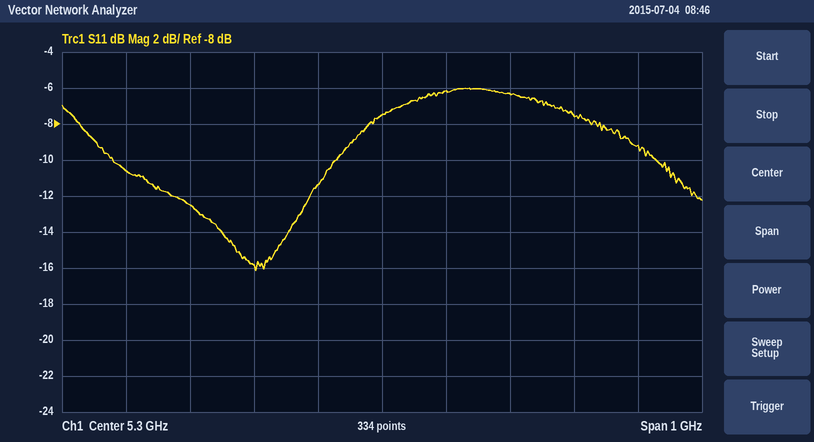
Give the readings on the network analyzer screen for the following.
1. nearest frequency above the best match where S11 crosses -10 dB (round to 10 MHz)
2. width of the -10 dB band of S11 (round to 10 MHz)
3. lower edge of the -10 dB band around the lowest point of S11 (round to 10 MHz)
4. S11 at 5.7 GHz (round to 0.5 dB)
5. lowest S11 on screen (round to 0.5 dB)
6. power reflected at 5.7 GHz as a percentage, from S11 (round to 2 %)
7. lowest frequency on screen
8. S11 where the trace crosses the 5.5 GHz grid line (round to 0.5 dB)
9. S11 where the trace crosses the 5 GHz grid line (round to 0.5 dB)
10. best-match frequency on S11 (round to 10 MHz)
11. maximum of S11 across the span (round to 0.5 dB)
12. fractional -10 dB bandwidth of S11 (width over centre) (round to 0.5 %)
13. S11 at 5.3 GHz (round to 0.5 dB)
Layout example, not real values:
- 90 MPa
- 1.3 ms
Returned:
- 5.23 GHz
- 350 MHz
- 4.88 GHz
- -9.0 dB
- -16.0 dB
- 12 %
- 4.8 GHz
- -6.5 dB
- -12.5 dB
- 5.10 GHz
- -6.0 dB
- 7.0 %
- -7.5 dB
